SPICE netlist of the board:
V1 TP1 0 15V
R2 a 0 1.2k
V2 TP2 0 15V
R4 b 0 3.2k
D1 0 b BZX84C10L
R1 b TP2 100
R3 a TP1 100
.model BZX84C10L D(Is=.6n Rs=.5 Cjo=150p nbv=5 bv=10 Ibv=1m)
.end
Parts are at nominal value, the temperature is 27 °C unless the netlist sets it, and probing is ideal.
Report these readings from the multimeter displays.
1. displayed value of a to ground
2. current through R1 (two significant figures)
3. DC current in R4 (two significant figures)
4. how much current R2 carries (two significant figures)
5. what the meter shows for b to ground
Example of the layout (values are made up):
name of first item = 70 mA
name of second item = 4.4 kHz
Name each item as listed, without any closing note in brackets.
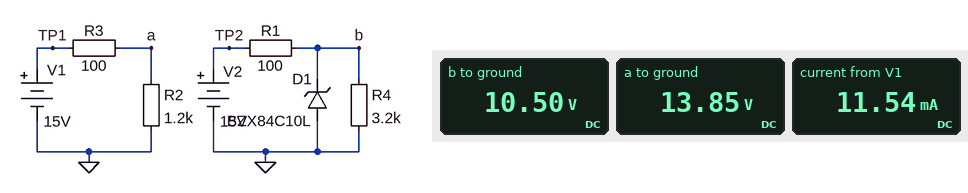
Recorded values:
displayed value of a to ground = 13.85 V
current through R1 = 45 mA
DC current in R4 = 3.3 mA
how much current R2 carries = 12 mA
what the meter shows for b to ground = 10.50 V
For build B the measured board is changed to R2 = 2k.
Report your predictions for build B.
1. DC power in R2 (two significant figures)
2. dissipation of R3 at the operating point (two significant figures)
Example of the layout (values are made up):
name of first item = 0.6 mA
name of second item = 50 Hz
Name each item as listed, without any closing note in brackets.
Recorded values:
DC power in R2 = 100 mW
dissipation of R3 at the operating point = 5.1 mW
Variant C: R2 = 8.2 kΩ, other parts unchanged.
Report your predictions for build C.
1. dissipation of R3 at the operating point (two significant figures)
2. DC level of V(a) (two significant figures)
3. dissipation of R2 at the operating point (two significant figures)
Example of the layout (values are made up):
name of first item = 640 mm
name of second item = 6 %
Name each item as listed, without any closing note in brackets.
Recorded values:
dissipation of R3 at the operating point = 330 µW
DC level of V(a) = 15 V
dissipation of R2 at the operating point = 27 mW
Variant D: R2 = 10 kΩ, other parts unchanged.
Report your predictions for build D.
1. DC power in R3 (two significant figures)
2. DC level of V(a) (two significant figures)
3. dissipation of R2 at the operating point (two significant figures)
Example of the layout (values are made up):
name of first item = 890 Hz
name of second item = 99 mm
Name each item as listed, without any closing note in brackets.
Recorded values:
DC power in R3 = 220 µW
DC level of V(a) = 15 V
dissipation of R2 at the operating point = 22 mW
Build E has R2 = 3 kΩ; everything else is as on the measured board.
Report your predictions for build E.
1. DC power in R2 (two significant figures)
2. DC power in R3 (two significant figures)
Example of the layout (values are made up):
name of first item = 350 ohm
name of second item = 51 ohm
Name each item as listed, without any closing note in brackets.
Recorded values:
DC power in R2 = 70 mW
DC power in R3 = 2.3 mW
